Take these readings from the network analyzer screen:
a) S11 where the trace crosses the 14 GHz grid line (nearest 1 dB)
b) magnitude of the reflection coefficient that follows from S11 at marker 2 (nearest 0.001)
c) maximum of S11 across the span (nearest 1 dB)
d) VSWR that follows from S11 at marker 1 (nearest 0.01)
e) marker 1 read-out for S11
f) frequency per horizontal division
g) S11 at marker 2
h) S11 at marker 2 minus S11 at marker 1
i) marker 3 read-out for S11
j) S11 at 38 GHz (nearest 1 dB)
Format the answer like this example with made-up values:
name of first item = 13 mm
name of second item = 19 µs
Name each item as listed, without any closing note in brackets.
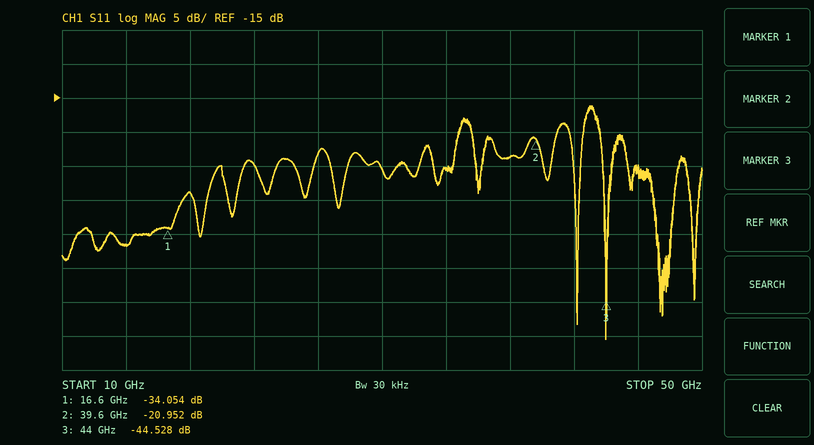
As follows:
S11 where the trace crosses the 14 GHz grid line = -37 dB
magnitude of the reflection coefficient that follows from S11 at marker 2 = 0.090
maximum of S11 across the span = -16 dB
VSWR that follows from S11 at marker 1 = 1.04
marker 1 read-out for S11 = -34.054 dB
frequency per horizontal division = 4 GHz
S11 at marker 2 = -20.952 dB
S11 at marker 2 minus S11 at marker 1 = 13.102 dB
marker 3 read-out for S11 = -44.528 dB
S11 at 38 GHz = -24 dB
